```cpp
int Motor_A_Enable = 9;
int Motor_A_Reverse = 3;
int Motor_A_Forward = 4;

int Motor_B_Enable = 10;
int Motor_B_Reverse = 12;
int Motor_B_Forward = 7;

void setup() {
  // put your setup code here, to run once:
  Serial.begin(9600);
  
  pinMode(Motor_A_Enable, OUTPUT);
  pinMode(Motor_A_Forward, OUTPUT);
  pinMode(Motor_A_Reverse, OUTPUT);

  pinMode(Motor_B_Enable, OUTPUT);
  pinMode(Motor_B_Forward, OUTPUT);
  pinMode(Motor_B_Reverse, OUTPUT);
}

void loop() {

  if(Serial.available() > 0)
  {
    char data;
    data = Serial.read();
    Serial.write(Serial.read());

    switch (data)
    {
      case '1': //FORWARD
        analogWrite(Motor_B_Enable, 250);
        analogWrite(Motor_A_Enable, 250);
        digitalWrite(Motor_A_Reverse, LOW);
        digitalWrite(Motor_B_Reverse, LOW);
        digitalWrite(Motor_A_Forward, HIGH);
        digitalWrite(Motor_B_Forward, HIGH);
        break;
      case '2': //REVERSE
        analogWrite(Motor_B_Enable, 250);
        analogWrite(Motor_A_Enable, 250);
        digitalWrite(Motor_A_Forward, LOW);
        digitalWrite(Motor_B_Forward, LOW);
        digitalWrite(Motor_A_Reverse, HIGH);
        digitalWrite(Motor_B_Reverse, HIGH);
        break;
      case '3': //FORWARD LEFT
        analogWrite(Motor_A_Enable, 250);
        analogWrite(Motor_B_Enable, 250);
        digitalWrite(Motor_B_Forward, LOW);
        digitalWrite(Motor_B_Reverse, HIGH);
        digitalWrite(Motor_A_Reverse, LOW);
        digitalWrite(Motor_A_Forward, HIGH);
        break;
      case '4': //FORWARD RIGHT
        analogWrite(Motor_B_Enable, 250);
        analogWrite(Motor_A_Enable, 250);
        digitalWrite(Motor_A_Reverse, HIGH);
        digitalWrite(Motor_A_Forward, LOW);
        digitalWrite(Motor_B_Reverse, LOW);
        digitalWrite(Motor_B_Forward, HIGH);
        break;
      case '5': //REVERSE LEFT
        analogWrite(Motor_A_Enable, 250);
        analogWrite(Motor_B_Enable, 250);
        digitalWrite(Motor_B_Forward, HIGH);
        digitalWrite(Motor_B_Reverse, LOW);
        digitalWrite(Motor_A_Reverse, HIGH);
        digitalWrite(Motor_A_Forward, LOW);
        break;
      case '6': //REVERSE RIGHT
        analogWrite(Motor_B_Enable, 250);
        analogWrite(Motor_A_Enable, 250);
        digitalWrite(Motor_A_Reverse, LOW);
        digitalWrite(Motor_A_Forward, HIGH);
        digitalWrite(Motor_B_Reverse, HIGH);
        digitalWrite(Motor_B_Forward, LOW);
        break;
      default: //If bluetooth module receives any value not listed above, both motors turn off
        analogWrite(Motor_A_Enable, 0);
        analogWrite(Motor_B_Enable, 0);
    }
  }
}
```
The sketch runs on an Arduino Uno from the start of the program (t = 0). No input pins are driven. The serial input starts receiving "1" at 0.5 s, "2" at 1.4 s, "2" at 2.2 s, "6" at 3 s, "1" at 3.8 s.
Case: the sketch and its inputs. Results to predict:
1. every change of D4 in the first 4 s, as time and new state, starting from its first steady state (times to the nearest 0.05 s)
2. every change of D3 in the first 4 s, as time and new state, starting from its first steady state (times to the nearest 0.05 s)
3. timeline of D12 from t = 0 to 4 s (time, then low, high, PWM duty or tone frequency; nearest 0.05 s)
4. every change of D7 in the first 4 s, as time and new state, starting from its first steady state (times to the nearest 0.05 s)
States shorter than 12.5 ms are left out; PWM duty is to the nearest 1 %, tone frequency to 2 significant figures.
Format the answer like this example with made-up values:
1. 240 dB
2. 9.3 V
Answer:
1. 0 s low; 0.5 s high; 1.4 s low; 3 s high
2. 0 s low; 1.4 s high; 3 s low
3. 0 s low; 1.4 s high; 3.8 s low
4. 0 s low; 0.5 s high; 1.4 s low; 3.8 s high
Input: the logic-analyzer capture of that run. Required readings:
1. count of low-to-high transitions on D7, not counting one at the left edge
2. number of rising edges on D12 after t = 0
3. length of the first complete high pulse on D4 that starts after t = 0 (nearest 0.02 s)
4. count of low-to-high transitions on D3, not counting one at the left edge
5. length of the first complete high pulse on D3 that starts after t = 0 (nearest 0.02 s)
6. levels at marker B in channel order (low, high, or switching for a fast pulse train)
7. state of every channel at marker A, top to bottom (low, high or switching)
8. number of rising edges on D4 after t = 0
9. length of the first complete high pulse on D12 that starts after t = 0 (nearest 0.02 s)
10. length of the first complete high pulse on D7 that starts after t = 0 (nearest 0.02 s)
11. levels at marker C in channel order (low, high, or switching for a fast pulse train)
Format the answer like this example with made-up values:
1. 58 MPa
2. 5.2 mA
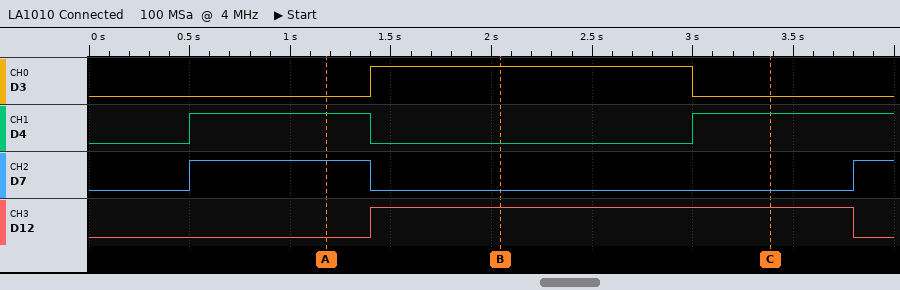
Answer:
1. 2
2. 1
3. 0.90 s
4. 1
5. 1.60 s
6. D3 high, D4 low, D7 low, D12 high
7. D3 low, D4 high, D7 high, D12 low
8. 2
9. 2.40 s
10. 0.90 s
11. D3 low, D4 high, D7 low, D12 high
